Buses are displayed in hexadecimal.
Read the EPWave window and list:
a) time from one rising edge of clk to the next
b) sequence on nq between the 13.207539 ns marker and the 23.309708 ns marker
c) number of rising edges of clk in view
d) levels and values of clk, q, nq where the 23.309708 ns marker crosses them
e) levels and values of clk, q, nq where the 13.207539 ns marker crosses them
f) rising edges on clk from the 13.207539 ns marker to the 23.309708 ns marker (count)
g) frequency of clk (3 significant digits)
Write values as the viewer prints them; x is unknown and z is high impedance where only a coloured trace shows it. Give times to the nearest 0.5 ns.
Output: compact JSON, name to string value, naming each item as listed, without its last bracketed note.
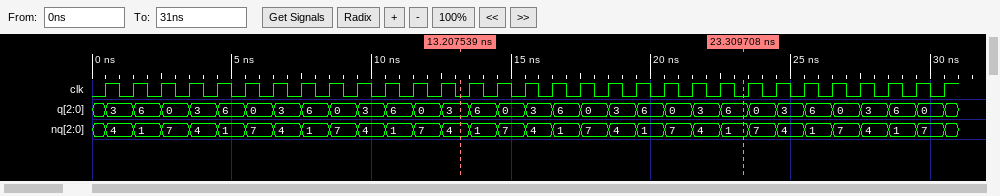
{"time from one rising edge of clk to the next": "1 ns", "sequence on nq between the 13.207539 ns marker and the 23.309708 ns marker": "4, 1, 7, 4, 1, 7, 4, 1, 7, 4, 1", "number of rising edges of clk in view": "31", "levels and values of clk, q, nq where the 23.309708 ns marker crosses them": "clk=0, q=6, nq=1", "levels and values of clk, q, nq where the 13.207539 ns marker crosses them": "clk=0, q=3, nq=4", "rising edges on clk from the 13.207539 ns marker to the 23.309708 ns marker": "10", "frequency of clk": "1.00 GHz"}
